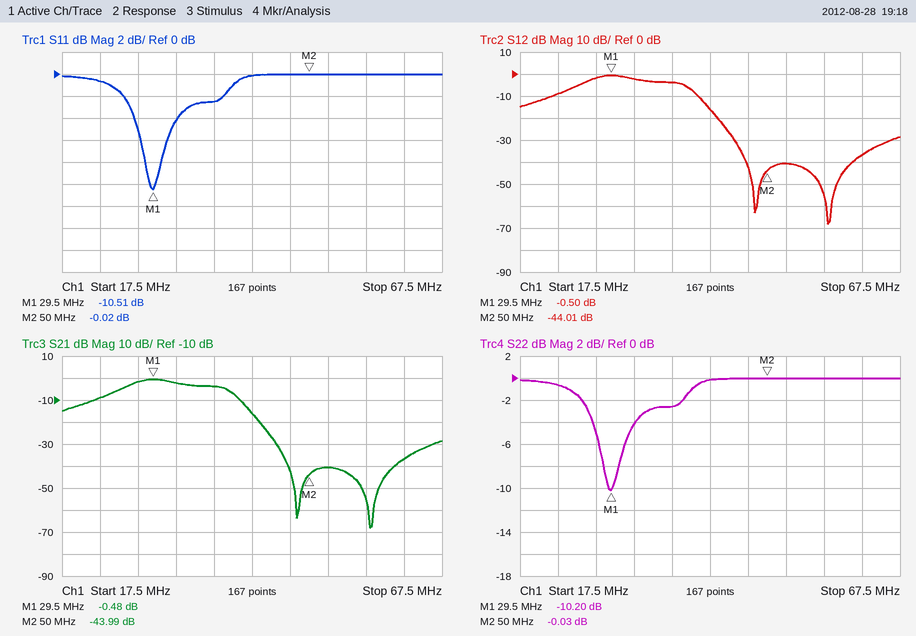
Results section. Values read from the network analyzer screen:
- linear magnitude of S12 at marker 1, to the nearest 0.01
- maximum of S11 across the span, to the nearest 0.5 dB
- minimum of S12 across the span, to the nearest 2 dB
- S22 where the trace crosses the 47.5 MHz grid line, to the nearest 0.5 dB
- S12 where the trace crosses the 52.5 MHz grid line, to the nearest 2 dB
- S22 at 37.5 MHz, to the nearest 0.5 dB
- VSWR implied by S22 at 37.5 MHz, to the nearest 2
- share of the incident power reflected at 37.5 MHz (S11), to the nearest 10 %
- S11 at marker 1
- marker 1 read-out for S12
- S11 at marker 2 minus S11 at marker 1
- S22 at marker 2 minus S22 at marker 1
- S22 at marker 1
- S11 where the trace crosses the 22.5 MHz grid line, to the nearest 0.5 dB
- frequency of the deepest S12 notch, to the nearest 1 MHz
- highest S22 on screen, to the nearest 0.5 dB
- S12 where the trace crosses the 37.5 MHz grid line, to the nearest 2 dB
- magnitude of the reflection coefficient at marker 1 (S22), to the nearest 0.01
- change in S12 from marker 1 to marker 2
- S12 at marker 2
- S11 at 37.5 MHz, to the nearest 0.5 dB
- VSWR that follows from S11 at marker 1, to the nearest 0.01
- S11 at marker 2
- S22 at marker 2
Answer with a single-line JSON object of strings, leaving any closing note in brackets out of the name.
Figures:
{"linear magnitude of S12 at marker 1, to the nearest 0.01": "0.94", "maximum of S11 across the span, to the nearest 0.5 dB": "0.0 dB", "minimum of S12 across the span, to the nearest 2 dB": "-68 dB", "S22 where the trace crosses the 47.5 MHz grid line, to the nearest 0.5 dB": "0.0 dB", "S12 where the trace crosses the 52.5 MHz grid line, to the nearest 2 dB": "-40 dB", "S22 at 37.5 MHz, to the nearest 0.5 dB": "-2.5 dB", "VSWR implied by S22 at 37.5 MHz, to the nearest 2": "6", "share of the incident power reflected at 37.5 MHz (S11), to the nearest 10 %": "60 %", "S11 at marker 1": "-10.51 dB", "marker 1 read-out for S12": "-0.50 dB", "S11 at marker 2 minus S11 at marker 1": "10.49 dB", "S22 at marker 2 minus S22 at marker 1": "10.17 dB", "S22 at marker 1": "-10.20 dB", "S11 where the trace crosses the 22.5 MHz grid line, to the nearest 0.5 dB": "-0.5 dB", "frequency of the deepest S12 notch, to the nearest 1 MHz": "58 MHz", "highest S22 on screen, to the nearest 0.5 dB": "0.0 dB", "S12 where the trace crosses the 37.5 MHz grid line, to the nearest 2 dB": "-4 dB", "magnitude of the reflection coefficient at marker 1 (S22), to the nearest 0.01": "0.31", "change in S12 from marker 1 to marker 2": "-43.51 dB", "S12 at marker 2": "-44.01 dB", "S11 at 37.5 MHz, to the nearest 0.5 dB": "-2.5 dB", "VSWR that follows from S11 at marker 1, to the nearest 0.01": "1.85", "S11 at marker 2": "-0.02 dB", "S22 at marker 2": "-0.03 dB"}
